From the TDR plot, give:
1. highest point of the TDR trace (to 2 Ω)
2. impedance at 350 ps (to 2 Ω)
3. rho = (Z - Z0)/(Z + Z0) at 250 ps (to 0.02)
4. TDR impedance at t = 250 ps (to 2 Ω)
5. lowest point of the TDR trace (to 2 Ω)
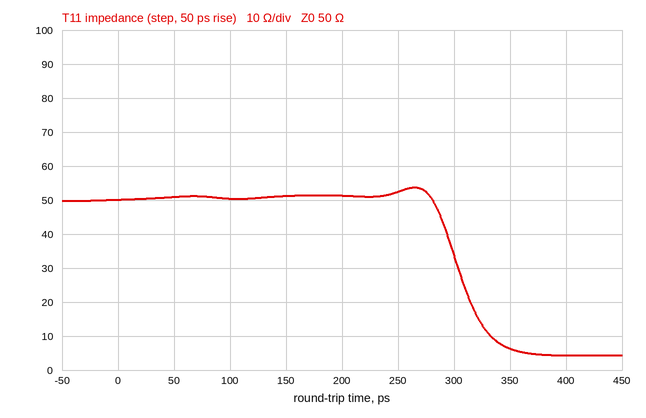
54 Ω
6 Ω
+0.02
52 Ω
4 Ω
